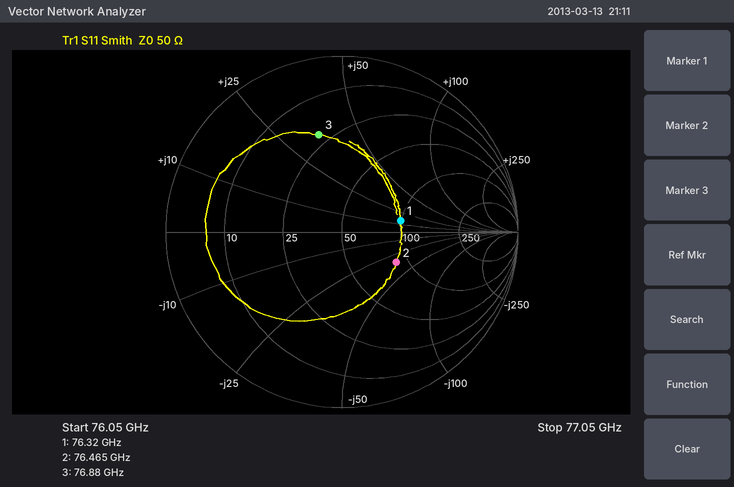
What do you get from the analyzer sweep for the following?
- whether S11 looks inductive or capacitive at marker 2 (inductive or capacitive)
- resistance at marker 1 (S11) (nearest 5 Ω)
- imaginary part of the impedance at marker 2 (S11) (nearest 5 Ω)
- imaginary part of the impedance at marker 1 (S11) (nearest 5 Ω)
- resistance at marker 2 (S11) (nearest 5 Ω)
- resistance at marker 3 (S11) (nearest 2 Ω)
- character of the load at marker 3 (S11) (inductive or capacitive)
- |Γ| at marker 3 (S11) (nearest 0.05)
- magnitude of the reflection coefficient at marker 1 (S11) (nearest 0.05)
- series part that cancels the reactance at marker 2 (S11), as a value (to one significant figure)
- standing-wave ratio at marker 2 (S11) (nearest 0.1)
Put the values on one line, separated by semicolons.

capacitive; 100 Ω; -35 Ω; +15 Ω; 85 Ω; 22 Ω; inductive; 0.55; 0.35; 70 pH; 2.1
